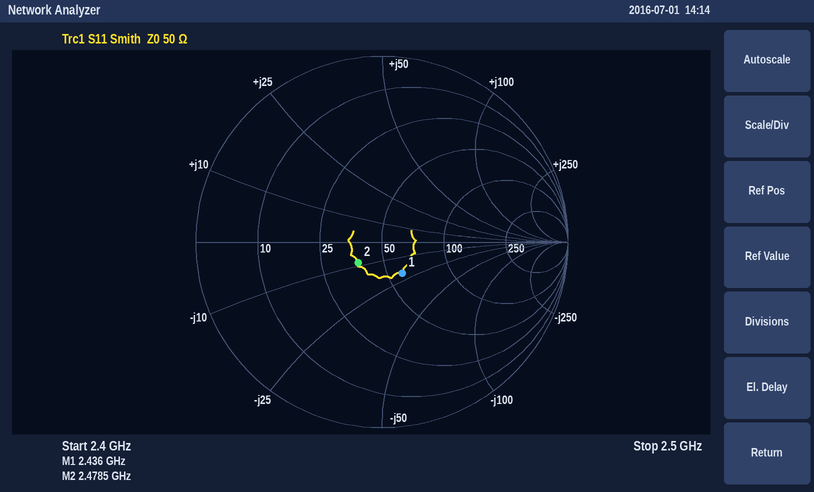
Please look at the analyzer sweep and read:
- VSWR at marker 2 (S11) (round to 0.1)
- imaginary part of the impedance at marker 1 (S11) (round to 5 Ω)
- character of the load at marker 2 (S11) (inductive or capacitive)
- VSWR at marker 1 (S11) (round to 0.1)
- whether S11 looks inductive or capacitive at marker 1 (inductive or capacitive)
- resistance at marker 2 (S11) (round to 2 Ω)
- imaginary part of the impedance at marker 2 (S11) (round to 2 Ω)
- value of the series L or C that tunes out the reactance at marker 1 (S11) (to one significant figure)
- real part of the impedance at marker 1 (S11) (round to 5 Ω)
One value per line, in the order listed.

1.4
-20 Ω
capacitive
1.5
capacitive
38 Ω
-8 Ω
1 nH
60 Ω
